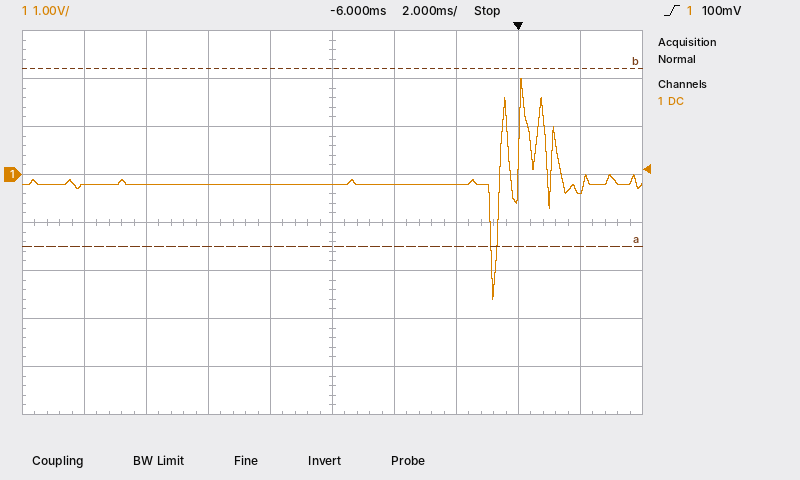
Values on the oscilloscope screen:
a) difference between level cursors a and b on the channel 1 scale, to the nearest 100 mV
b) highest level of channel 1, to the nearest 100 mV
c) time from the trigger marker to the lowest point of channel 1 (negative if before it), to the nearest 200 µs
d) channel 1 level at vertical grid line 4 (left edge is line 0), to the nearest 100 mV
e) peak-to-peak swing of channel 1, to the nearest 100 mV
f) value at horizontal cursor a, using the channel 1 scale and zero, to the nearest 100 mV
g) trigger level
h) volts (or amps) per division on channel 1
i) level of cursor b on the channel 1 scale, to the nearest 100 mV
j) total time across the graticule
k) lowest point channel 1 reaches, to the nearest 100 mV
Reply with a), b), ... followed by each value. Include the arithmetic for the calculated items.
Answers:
a) 3.7 V
b) 2.0 V
c) -800 µs
d) -200 mV
e) 2.0 V − (-2.6 V) = 4.6 V
f) -1.5 V
g) 100 mV
h) 1 V
i) 2.2 V
j) 20 ms
k) -2.6 V
